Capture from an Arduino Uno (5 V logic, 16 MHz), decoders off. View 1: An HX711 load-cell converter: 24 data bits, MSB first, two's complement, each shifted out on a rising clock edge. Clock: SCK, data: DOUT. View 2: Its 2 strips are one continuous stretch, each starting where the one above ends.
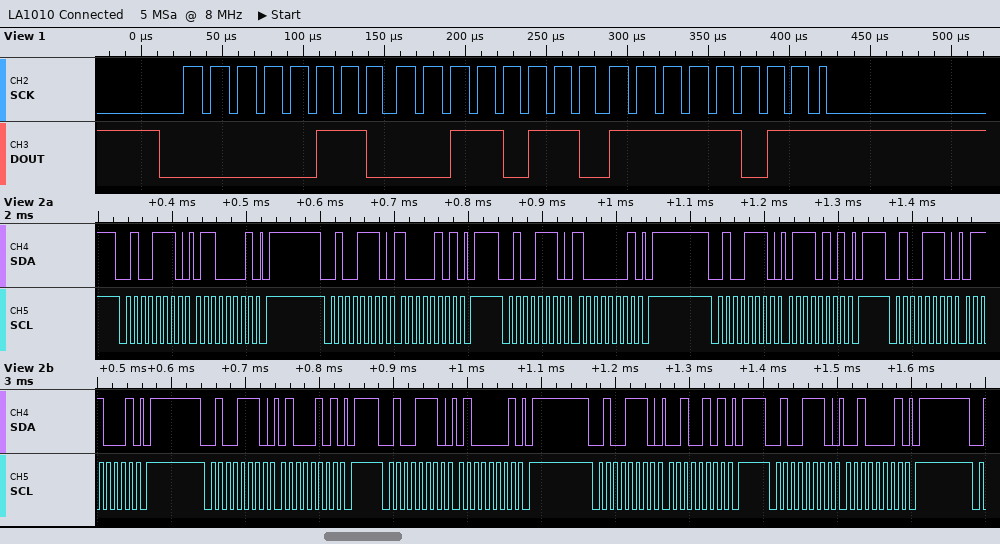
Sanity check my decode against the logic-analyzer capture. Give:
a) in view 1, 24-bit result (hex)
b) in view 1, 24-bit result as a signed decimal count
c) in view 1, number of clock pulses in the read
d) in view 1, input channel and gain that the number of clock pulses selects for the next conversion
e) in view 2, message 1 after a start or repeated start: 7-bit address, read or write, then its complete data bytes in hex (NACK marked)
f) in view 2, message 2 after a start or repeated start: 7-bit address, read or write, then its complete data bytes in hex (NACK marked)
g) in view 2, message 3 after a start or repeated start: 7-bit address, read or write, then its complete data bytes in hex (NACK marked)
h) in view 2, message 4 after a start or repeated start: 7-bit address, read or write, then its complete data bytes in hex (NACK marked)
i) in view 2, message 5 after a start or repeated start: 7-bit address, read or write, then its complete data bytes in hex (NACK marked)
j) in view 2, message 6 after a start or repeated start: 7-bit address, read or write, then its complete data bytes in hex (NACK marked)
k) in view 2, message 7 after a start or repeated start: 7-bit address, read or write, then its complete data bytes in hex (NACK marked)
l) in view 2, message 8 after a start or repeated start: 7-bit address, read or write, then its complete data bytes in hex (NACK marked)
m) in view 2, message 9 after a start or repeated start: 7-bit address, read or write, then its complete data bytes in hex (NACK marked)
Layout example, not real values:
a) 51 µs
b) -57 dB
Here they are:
a) 0x0636FB
b) 407291
c) 25
d) channel A, gain 128
e) 0x27 write: 61
f) 0x27 write: 85
g) 0x27 write: 81
h) 0x27 write: 75
i) 0x27 write: 71
j) 0x27 write: 45
k) 0x27 write: 41
l) 0x27 write: 25
m) 0x27 write: 21
